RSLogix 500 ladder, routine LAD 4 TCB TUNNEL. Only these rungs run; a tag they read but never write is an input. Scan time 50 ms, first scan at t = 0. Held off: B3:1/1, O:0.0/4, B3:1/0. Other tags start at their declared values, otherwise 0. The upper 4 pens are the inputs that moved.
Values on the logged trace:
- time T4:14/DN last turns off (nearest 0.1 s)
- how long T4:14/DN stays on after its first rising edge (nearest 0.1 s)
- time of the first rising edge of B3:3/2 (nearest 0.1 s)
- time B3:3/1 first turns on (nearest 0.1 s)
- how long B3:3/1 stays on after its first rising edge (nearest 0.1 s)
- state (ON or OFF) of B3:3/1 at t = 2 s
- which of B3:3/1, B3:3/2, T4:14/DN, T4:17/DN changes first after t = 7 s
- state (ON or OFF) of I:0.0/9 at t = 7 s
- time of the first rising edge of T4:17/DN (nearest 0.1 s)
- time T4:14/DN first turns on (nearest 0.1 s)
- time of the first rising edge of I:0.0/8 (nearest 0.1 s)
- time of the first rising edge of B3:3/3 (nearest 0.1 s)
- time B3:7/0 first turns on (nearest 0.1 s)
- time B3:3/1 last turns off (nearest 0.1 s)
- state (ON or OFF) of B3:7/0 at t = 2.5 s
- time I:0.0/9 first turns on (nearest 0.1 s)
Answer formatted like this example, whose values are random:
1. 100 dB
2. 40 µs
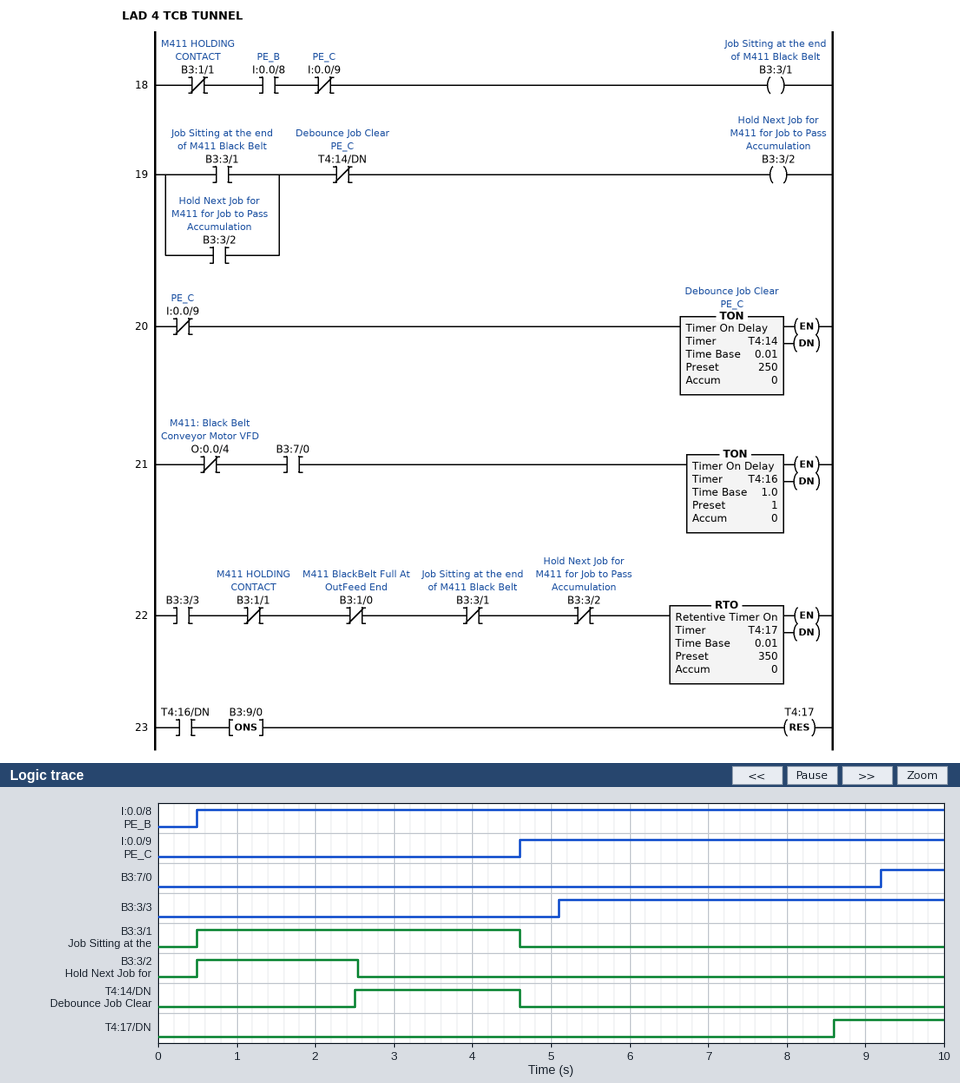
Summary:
1. 4.6 s
2. 2.1 s
3. 0.5 s
4. 0.5 s
5. 4.1 s
6. ON
7. T4:17/DN
8. ON
9. 8.6 s
10. 2.5 s
11. 0.5 s
12. 5.1 s
13. 9.2 s
14. 4.6 s
15. OFF
16. 4.6 s
